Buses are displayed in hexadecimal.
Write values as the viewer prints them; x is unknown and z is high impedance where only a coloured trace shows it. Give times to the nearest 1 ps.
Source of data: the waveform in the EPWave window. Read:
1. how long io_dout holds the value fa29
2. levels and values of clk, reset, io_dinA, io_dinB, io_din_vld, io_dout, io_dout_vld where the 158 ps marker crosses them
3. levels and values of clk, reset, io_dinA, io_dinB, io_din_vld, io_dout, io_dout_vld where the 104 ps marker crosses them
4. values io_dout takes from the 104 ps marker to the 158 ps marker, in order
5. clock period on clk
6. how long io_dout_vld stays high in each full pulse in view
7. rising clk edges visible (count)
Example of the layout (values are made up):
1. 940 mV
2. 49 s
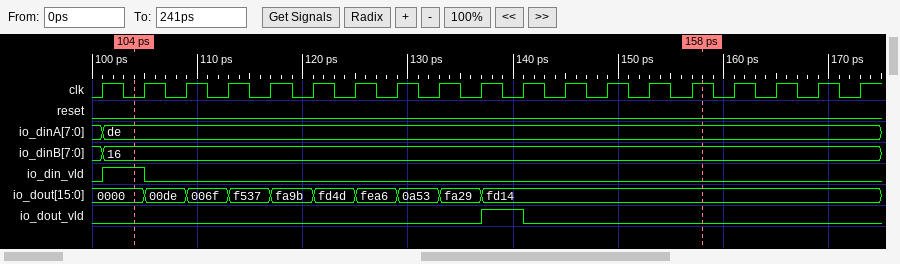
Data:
1. 4 ps
2. clk=1, reset=0, io_dinA=de, io_dinB=16, io_din_vld=0, io_dout=fd14, io_dout_vld=0
3. clk=0, reset=0, io_dinA=de, io_dinB=16, io_din_vld=1, io_dout=0000, io_dout_vld=0
4. 0000, 00de, 006f, f537, fa9b, fd4d, fea6, 0a53, fa29, fd14
5. 4 ps
6. 4 ps
7. 19
